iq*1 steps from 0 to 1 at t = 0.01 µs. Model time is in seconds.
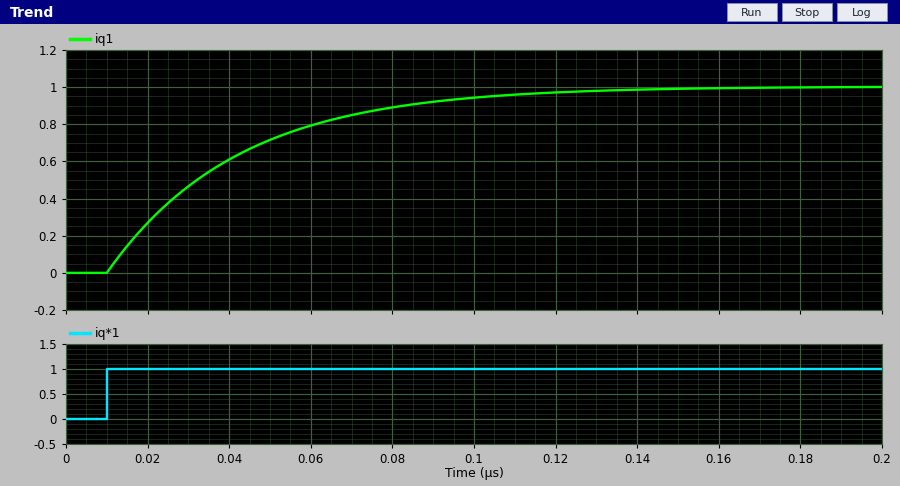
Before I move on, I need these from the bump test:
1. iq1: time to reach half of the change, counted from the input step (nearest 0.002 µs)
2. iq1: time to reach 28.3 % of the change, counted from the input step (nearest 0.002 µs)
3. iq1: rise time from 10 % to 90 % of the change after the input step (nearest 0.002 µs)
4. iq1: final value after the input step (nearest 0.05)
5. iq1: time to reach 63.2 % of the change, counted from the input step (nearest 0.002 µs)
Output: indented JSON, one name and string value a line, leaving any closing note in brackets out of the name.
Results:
{
  "iq1: time to reach half of the change, counted from the input step": "0.022 µs",
  "iq1: time to reach 28.3 % of the change, counted from the input step": "0.010 µs",
  "iq1: rise time from 10 % to 90 % of the change after the input step": "0.070 µs",
  "iq1: final value after the input step": "1.00",
  "iq1: time to reach 63.2 % of the change, counted from the input step": "0.032 µs"
}
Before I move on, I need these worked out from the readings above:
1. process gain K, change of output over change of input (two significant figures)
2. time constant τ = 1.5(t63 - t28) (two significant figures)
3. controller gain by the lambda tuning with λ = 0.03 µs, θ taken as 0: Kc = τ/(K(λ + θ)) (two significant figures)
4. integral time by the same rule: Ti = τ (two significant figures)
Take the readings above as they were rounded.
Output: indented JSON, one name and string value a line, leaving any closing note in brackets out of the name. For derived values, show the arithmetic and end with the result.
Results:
{
  "process gain K, change of output over change of input": "(1 - 0) / 1 = 1.0",
  "time constant τ = 1.5(t63 - t28)": "1.5 × (0.032 - 0.01) = 0.033 µs",
  "controller gain by the lambda tuning with λ = 0.03 µs, θ taken as 0: Kc = τ/(K(λ + θ))": "0.033 / (1 × (0.03 + 0)) = 1.1",
  "integral time by the same rule: Ti = τ": "0.033 µs"
}
